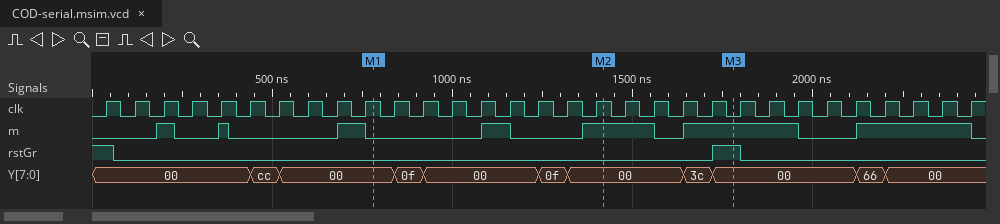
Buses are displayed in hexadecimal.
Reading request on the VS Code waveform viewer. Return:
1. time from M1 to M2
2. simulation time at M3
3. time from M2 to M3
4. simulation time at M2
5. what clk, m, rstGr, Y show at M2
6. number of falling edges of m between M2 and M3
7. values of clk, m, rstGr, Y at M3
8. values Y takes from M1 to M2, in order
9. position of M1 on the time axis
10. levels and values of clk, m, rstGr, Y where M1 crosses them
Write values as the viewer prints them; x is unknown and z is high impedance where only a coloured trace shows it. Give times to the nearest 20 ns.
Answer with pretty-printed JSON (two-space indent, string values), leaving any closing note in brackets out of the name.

{
  "time from M1 to M2": "640 ns",
  "simulation time at M3": "1780 ns",
  "time from M2 to M3": "360 ns",
  "simulation time at M2": "1420 ns",
  "what clk, m, rstGr, Y show at M2": "clk=1, m=1, rstGr=0, Y=00",
  "number of falling edges of m between M2 and M3": "1",
  "values of clk, m, rstGr, Y at M3": "clk=0, m=1, rstGr=1, Y=00",
  "values Y takes from M1 to M2, in order": "00, 0f, 00, 0f, 00",
  "position of M1 on the time axis": "780 ns",
  "levels and values of clk, m, rstGr, Y where M1 crosses them": "clk=1, m=0, rstGr=0, Y=00"
}
